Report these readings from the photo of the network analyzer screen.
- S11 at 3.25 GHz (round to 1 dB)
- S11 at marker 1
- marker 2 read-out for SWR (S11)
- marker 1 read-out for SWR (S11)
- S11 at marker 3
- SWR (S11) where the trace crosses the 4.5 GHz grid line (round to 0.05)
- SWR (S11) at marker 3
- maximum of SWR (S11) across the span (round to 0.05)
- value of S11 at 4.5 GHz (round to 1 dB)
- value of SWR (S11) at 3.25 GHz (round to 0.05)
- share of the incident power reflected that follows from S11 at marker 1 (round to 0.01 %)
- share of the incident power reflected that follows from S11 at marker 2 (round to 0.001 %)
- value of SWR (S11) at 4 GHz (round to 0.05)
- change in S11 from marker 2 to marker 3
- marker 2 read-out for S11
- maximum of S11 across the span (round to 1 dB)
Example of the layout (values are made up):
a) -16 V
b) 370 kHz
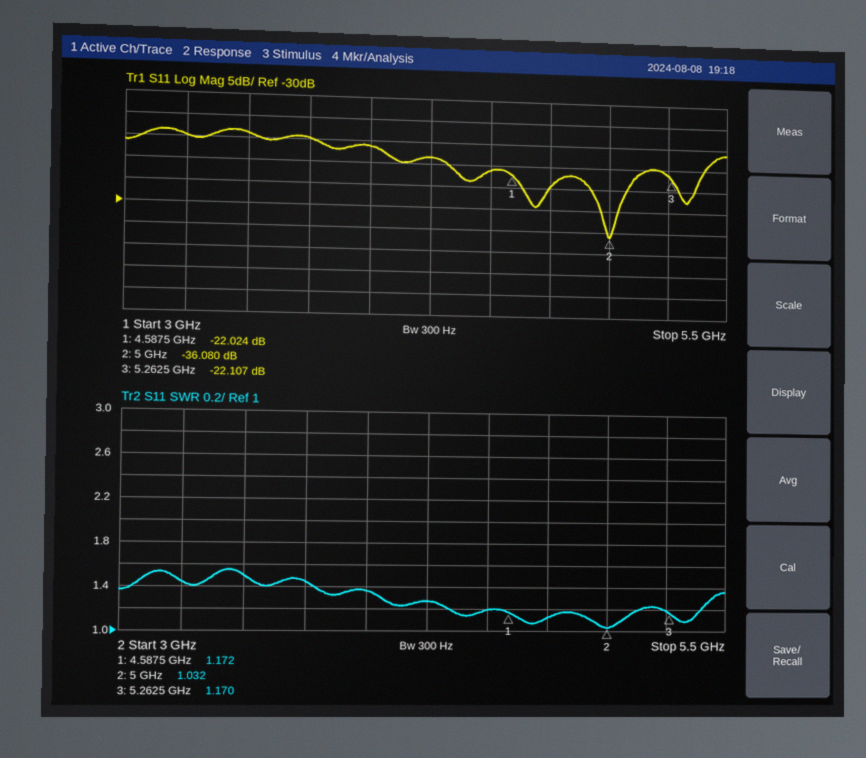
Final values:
a) -15 dB
b) -22.024 dB
c) 1.032
d) 1.172
e) -22.107 dB
f) 1.20
g) 1.170
h) 1.55
i) -21 dB
j) 1.45
k) 0.63 %
l) 0.025 %
m) 1.35
n) 13.973 dB
o) -36.080 dB
p) -13 dB
